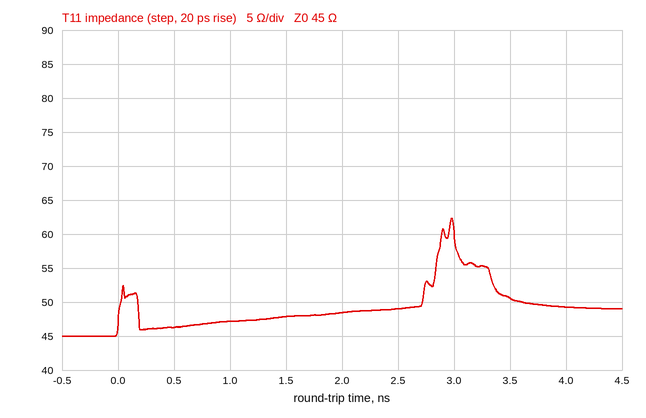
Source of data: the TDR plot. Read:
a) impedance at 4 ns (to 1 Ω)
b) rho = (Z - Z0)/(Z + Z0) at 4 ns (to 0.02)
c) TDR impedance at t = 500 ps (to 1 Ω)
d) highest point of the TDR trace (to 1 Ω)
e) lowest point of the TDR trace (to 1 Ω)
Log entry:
49 Ω
+0.04
46 Ω
62 Ω
45 Ω
